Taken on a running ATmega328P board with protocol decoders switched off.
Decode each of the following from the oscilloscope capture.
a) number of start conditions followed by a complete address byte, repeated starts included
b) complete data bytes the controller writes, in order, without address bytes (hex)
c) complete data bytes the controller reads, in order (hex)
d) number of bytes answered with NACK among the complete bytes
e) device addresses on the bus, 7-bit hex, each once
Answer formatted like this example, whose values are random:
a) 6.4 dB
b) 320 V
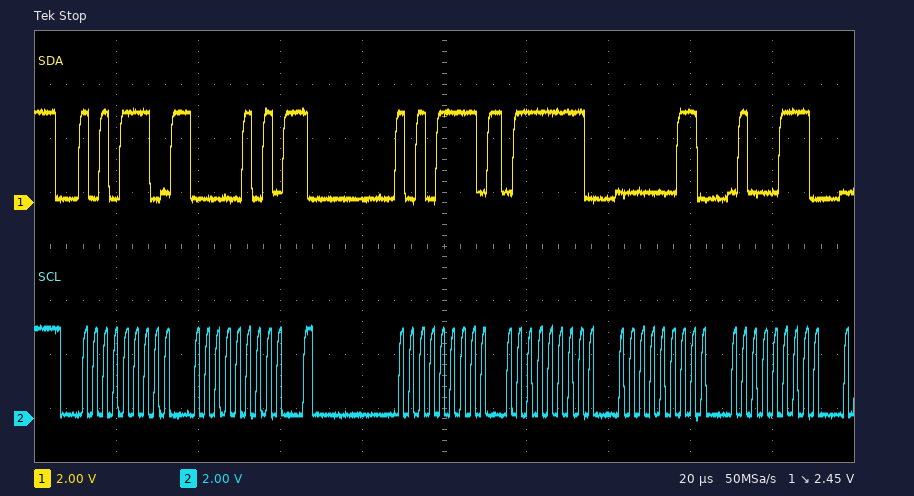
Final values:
a) 2
b) 05
c) 7F 03 47
d) 0
e) 0x57
